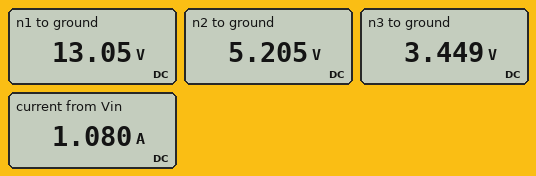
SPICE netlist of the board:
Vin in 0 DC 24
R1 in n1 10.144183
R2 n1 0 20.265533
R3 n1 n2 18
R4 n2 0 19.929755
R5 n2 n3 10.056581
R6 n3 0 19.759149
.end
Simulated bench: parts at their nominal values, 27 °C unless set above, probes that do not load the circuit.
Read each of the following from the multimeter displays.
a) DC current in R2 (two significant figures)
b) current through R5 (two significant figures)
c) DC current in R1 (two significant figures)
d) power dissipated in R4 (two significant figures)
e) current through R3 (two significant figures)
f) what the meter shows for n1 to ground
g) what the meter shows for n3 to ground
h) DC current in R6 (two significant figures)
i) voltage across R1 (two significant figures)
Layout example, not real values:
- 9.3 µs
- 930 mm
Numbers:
- 640 mA
- 170 mA
- 1.1 A
- 1.4 W
- 440 mA
- 13.05 V
- 3.449 V
- 170 mA
- 11 V
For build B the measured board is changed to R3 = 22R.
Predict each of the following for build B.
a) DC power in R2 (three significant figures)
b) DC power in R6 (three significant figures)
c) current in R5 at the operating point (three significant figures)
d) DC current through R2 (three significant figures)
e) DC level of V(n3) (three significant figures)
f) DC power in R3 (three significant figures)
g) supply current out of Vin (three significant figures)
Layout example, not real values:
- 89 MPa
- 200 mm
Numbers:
- 8.78 W
- 490 mW
- 157 mA
- 658 mA
- 3.11 V
- 3.40 W
- 1.05 A
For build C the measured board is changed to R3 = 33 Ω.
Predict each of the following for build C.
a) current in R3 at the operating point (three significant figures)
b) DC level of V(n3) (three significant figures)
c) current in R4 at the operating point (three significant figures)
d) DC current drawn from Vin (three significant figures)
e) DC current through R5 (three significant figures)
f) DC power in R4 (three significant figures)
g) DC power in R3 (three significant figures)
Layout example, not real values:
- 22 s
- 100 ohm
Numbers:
- 309 mA
- 2.45 V
- 185 mA
- 995 mA
- 124 mA
- 685 mW
- 3.16 W
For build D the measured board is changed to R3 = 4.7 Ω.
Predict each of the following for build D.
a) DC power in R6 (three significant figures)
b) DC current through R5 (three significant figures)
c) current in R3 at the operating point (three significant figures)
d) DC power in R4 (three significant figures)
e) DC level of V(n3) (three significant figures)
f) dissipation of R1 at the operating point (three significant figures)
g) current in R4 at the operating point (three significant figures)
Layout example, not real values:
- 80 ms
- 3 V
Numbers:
- 1.48 W
- 274 mA
- 683 mA
- 3.34 W
- 5.41 V
- 15.7 W
- 410 mA
